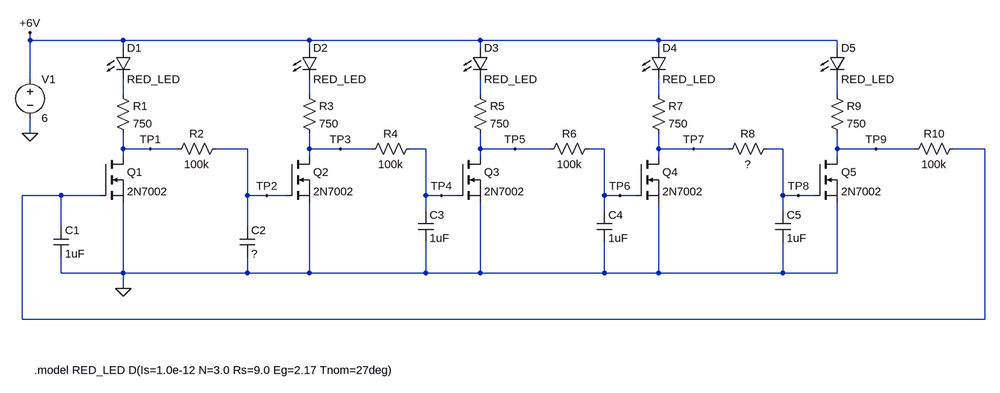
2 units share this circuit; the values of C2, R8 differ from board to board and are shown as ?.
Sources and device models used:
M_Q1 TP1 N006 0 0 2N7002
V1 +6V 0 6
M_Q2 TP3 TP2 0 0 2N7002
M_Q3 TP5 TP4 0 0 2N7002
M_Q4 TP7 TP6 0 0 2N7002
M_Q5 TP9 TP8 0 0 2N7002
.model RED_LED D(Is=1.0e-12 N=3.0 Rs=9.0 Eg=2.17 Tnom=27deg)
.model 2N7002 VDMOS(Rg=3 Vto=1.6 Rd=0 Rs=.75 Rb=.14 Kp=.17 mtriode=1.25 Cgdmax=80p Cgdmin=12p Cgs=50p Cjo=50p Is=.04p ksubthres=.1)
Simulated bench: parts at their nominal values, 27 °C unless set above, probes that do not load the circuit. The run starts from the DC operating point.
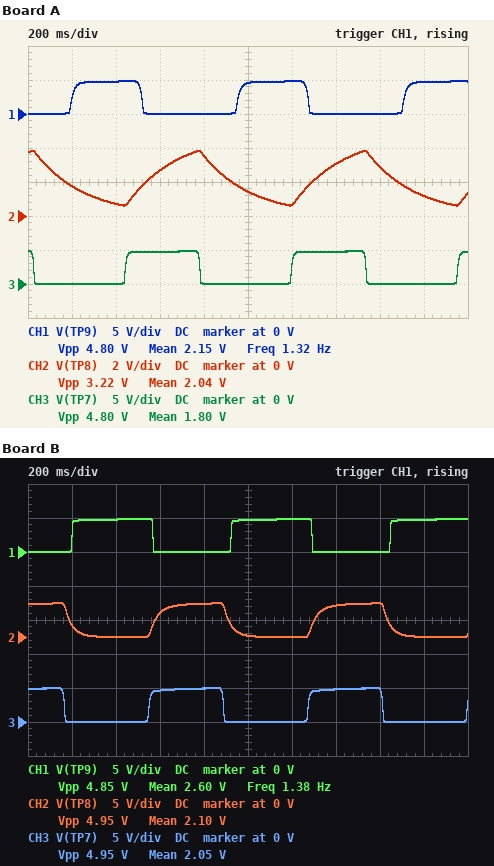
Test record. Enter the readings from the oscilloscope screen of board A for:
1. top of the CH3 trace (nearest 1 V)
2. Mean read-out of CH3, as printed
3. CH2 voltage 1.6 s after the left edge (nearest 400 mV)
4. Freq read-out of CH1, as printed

5 V
1.80 V
2.8 V
1.32 Hz
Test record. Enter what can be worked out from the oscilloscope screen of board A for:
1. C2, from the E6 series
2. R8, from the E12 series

470 nF
220 kΩ
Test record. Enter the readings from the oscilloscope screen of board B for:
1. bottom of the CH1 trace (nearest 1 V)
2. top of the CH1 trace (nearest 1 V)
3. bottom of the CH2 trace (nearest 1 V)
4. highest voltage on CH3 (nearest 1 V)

0 V
5 V
0 V
5 V
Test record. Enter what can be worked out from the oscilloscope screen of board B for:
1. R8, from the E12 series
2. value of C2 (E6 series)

33 kΩ
2.2 µF
